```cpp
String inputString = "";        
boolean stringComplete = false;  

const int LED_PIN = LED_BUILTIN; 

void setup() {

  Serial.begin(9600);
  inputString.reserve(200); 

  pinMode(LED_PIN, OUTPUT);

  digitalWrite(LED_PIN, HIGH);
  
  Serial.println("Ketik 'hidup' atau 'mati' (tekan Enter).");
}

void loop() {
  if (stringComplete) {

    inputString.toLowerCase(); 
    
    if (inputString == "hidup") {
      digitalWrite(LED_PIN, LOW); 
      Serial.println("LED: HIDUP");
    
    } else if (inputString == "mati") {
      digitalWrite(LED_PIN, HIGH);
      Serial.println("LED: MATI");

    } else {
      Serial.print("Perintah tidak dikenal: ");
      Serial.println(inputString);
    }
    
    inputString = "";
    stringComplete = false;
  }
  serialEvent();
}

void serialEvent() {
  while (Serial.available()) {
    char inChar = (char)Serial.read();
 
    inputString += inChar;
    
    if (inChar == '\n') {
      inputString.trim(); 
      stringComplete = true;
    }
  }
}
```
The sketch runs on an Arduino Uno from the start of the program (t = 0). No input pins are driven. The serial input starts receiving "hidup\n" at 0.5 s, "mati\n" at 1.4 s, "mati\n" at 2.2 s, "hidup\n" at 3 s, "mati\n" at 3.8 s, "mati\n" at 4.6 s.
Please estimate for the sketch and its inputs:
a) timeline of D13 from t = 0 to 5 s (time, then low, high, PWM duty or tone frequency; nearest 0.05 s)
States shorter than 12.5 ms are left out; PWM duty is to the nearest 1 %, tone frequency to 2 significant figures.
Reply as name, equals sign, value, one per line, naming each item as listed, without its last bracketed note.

timeline of D13 from t = 0 to 5 s = 0 s high; 0.5 s low; 1.4 s high; 3 s low; 3.8 s high
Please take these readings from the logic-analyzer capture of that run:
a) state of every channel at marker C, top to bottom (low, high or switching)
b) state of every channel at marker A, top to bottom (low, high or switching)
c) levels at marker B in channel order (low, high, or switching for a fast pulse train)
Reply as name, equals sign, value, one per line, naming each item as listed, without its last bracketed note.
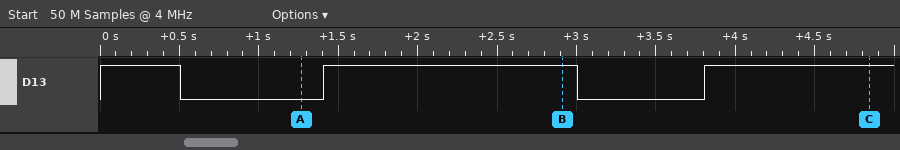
state of every channel at marker C, top to bottom = D13 high
state of every channel at marker A, top to bottom = D13 low
levels at marker B in channel order = D13 high
